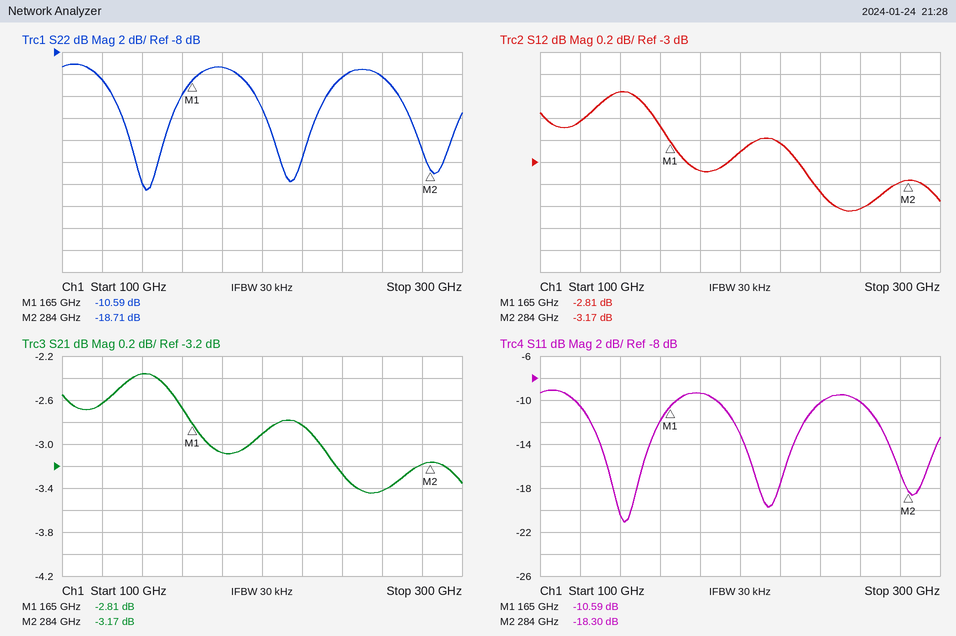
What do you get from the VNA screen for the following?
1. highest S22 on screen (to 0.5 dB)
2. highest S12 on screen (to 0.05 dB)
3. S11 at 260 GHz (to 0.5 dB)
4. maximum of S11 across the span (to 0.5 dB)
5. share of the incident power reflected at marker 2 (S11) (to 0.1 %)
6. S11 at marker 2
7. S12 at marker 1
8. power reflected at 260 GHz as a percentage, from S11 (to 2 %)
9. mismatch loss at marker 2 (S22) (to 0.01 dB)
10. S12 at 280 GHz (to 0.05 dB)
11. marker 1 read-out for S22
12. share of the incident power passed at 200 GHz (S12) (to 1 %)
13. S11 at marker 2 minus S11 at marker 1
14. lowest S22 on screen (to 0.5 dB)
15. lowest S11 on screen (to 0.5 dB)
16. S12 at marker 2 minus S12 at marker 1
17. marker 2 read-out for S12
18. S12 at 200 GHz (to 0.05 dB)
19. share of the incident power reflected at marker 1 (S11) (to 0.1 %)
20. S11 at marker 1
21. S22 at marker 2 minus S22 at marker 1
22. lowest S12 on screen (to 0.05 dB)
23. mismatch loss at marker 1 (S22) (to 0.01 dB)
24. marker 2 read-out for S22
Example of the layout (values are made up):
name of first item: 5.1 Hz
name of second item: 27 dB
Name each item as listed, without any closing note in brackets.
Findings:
highest S22 on screen: -9.0 dB
highest S12 on screen: -2.35 dB
S11 at 260 GHz: -10.0 dB
maximum of S11 across the span: -9.0 dB
share of the incident power reflected at marker 2 (S11): 1.5 %
S11 at marker 2: -18.30 dB
S12 at marker 1: -2.81 dB
power reflected at 260 GHz as a percentage, from S11: 10 %
mismatch loss at marker 2 (S22): 0.06 dB
S12 at 280 GHz: -3.20 dB
marker 1 read-out for S22: -10.59 dB
share of the incident power passed at 200 GHz (S12): 51 %
S11 at marker 2 minus S11 at marker 1: -7.71 dB
lowest S22 on screen: -20.5 dB
lowest S11 on screen: -21.0 dB
S12 at marker 2 minus S12 at marker 1: -0.36 dB
marker 2 read-out for S12: -3.17 dB
S12 at 200 GHz: -2.90 dB
share of the incident power reflected at marker 1 (S11): 8.7 %
S11 at marker 1: -10.59 dB
S22 at marker 2 minus S22 at marker 1: -8.12 dB
lowest S12 on screen: -3.45 dB
mismatch loss at marker 1 (S22): 0.40 dB
marker 2 read-out for S22: -18.71 dB
